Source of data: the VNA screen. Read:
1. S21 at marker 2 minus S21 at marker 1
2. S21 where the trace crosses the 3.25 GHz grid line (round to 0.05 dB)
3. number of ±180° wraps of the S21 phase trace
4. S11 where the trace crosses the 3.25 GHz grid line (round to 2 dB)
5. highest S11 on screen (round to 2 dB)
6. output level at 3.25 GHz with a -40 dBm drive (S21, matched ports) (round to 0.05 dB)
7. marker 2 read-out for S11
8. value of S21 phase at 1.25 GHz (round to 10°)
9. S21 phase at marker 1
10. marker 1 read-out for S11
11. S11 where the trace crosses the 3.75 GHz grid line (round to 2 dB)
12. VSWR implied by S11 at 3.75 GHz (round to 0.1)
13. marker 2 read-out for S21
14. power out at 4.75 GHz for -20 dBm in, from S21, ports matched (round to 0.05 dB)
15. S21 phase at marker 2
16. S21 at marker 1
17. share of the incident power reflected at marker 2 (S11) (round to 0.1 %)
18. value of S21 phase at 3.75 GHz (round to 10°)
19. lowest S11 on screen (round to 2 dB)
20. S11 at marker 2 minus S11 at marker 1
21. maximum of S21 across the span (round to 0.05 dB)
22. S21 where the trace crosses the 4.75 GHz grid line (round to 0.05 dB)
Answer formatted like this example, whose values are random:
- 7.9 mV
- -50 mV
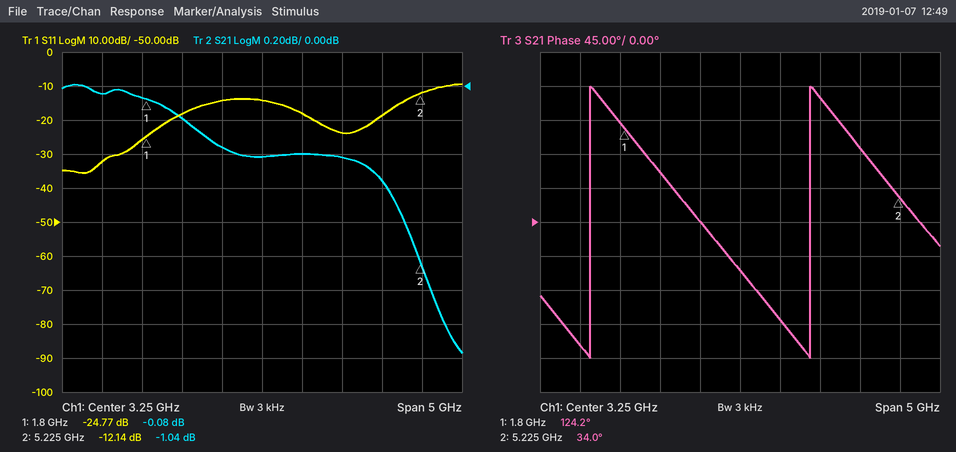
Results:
- -0.96 dB
- -0.40 dB
- 2
- -14 dB
- -10 dB
- -40.40 dBm
- -12.14 dB
- -160°
- 124.2°
- -24.77 dB
- -18 dB
- 1.3
- -1.04 dB
- -20.55 dBm
- 34.0°
- -0.08 dB
- 6.1 %
- -130°
- -36 dB
- 12.63 dB
- 0.00 dB
- -0.55 dB
